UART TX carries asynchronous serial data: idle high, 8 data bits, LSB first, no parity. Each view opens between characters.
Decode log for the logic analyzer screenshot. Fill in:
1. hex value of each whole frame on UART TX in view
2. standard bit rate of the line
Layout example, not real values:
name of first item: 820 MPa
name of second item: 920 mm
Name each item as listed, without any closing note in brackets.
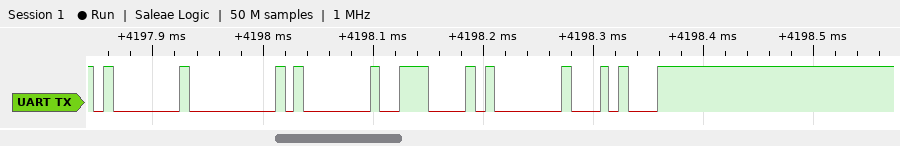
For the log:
hex value of each whole frame on UART TX in view: 01, 00, 01, 0E, 01, 14
standard bit rate of the line: 115200 baud
